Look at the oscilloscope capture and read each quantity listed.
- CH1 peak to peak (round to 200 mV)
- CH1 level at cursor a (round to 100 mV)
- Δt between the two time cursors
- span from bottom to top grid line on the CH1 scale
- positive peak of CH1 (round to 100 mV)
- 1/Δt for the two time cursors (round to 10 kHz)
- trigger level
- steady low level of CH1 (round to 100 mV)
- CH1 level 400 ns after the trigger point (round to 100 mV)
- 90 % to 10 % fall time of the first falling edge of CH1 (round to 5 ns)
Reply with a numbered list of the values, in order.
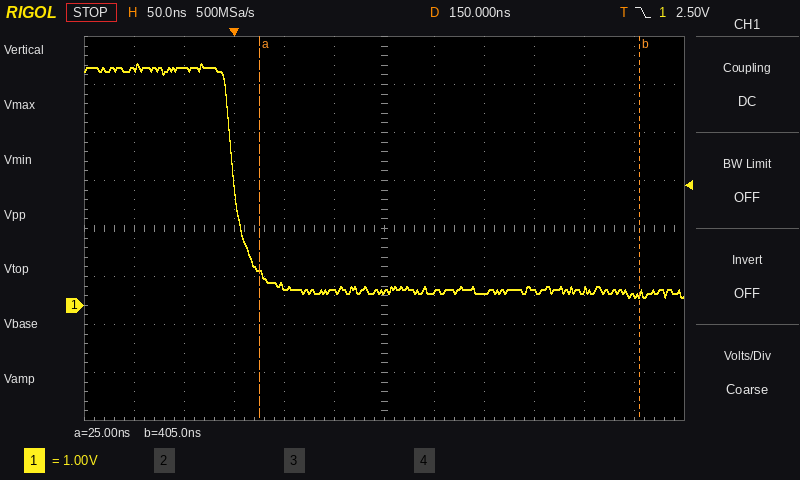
1. 4.8 V
2. 700 mV
3. 380 ns
4. 8 V
5. 5.0 V
6. 2.63 MHz
7. 2.50 V
8. 300 mV
9. 200 mV
10. 30 ns
